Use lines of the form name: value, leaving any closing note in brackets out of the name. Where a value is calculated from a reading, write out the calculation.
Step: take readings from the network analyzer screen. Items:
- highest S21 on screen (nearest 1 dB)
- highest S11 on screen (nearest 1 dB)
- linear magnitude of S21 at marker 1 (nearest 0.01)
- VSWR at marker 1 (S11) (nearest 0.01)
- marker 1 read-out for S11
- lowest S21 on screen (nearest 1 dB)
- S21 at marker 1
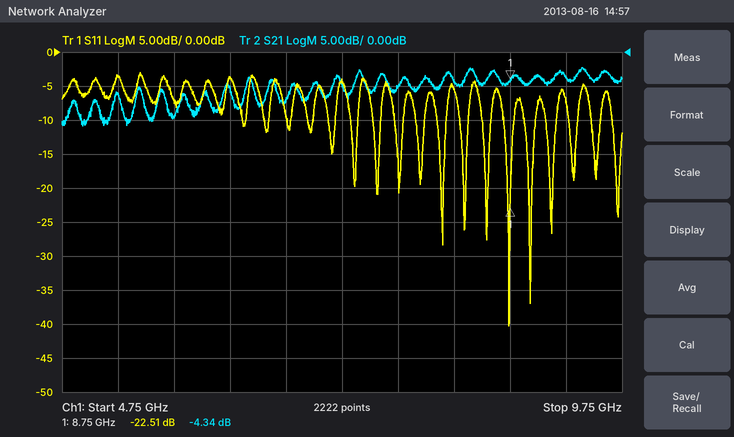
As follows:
highest S21 on screen: -2 dB
highest S11 on screen: -3 dB
linear magnitude of S21 at marker 1: 10^(-4.34/20) ≈ 0.61
VSWR at marker 1 (S11): (1 + 0.0749)/(1 − 0.0749) ≈ 1.16
marker 1 read-out for S11: -22.51 dB
lowest S21 on screen: -11 dB
S21 at marker 1: -4.34 dB
